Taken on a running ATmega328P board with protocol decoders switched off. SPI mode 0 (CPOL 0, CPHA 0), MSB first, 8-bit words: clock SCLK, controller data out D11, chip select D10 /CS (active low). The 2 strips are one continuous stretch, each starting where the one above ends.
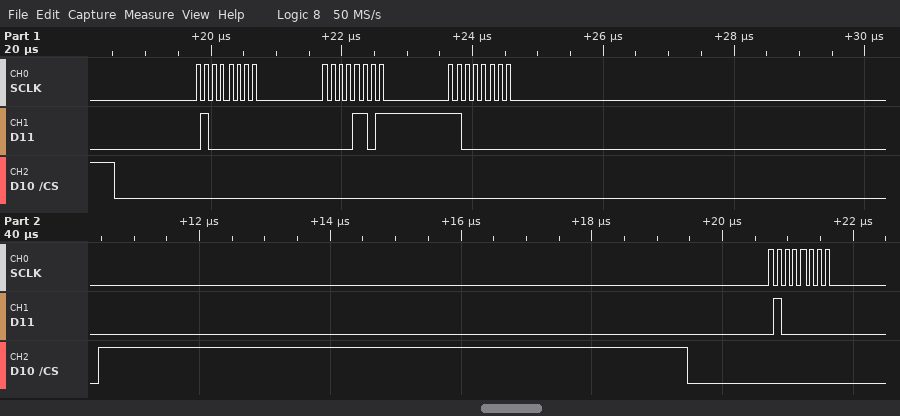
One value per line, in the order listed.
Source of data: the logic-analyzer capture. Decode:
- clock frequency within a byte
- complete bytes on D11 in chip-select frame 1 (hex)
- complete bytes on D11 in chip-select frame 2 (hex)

8 MHz
0x40 0x0D 0xC0
0x40
